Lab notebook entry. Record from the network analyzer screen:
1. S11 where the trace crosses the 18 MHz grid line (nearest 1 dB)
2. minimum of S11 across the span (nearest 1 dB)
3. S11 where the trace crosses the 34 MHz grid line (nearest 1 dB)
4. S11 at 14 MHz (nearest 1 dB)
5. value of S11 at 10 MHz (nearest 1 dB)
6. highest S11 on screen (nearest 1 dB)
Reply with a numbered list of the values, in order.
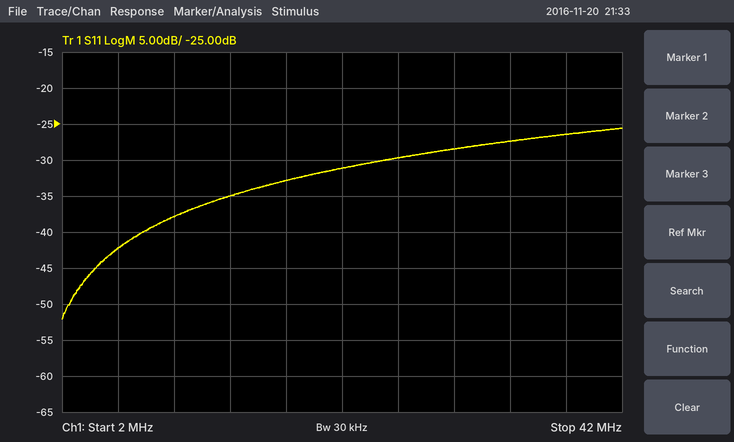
1. -33 dB
2. -52 dB
3. -27 dB
4. -35 dB
5. -38 dB
6. -26 dB
